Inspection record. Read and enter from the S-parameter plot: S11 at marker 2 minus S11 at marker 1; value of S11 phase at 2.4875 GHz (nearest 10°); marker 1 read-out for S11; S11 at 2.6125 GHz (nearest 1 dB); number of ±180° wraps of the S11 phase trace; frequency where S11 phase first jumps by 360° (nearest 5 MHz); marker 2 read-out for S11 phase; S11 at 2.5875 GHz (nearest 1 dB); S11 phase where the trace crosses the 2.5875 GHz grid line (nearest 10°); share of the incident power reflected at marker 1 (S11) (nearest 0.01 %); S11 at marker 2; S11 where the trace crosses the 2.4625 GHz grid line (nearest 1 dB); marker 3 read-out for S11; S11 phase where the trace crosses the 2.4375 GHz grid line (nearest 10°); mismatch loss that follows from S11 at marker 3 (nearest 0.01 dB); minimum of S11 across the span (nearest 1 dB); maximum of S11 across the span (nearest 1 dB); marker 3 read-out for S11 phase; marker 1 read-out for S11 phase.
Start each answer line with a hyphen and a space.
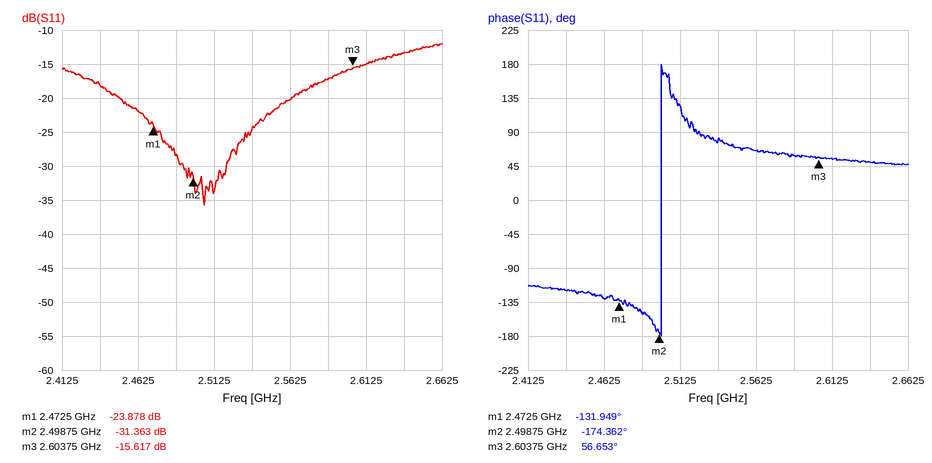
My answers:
- -7.485 dB
- -150°
- -23.878 dB
- -15 dB
- 1
- 2.500 GHz
- -174.362°
- -17 dB
- 60°
- 0.41 %
- -31.363 dB
- -22 dB
- -15.617 dB
- -120°
- 0.12 dB
- -36 dB
- -12 dB
- 56.653°
- -131.949°
